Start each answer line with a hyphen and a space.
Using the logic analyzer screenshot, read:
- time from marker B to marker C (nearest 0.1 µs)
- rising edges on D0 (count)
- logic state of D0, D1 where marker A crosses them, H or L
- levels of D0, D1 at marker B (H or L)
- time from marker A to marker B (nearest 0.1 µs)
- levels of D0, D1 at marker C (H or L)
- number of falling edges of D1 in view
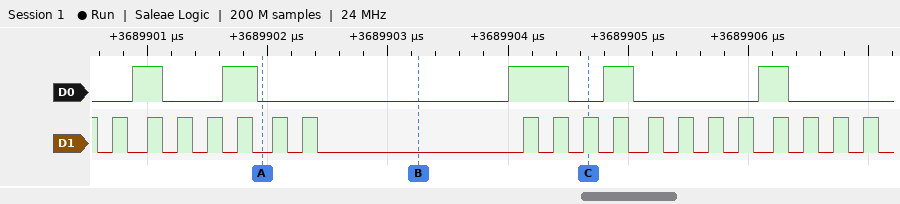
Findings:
- 1.4 µs
- 5
- D0=L, D1=L
- D0=L, D1=L
- 1.3 µs
- D0=L, D1=H
- 20
